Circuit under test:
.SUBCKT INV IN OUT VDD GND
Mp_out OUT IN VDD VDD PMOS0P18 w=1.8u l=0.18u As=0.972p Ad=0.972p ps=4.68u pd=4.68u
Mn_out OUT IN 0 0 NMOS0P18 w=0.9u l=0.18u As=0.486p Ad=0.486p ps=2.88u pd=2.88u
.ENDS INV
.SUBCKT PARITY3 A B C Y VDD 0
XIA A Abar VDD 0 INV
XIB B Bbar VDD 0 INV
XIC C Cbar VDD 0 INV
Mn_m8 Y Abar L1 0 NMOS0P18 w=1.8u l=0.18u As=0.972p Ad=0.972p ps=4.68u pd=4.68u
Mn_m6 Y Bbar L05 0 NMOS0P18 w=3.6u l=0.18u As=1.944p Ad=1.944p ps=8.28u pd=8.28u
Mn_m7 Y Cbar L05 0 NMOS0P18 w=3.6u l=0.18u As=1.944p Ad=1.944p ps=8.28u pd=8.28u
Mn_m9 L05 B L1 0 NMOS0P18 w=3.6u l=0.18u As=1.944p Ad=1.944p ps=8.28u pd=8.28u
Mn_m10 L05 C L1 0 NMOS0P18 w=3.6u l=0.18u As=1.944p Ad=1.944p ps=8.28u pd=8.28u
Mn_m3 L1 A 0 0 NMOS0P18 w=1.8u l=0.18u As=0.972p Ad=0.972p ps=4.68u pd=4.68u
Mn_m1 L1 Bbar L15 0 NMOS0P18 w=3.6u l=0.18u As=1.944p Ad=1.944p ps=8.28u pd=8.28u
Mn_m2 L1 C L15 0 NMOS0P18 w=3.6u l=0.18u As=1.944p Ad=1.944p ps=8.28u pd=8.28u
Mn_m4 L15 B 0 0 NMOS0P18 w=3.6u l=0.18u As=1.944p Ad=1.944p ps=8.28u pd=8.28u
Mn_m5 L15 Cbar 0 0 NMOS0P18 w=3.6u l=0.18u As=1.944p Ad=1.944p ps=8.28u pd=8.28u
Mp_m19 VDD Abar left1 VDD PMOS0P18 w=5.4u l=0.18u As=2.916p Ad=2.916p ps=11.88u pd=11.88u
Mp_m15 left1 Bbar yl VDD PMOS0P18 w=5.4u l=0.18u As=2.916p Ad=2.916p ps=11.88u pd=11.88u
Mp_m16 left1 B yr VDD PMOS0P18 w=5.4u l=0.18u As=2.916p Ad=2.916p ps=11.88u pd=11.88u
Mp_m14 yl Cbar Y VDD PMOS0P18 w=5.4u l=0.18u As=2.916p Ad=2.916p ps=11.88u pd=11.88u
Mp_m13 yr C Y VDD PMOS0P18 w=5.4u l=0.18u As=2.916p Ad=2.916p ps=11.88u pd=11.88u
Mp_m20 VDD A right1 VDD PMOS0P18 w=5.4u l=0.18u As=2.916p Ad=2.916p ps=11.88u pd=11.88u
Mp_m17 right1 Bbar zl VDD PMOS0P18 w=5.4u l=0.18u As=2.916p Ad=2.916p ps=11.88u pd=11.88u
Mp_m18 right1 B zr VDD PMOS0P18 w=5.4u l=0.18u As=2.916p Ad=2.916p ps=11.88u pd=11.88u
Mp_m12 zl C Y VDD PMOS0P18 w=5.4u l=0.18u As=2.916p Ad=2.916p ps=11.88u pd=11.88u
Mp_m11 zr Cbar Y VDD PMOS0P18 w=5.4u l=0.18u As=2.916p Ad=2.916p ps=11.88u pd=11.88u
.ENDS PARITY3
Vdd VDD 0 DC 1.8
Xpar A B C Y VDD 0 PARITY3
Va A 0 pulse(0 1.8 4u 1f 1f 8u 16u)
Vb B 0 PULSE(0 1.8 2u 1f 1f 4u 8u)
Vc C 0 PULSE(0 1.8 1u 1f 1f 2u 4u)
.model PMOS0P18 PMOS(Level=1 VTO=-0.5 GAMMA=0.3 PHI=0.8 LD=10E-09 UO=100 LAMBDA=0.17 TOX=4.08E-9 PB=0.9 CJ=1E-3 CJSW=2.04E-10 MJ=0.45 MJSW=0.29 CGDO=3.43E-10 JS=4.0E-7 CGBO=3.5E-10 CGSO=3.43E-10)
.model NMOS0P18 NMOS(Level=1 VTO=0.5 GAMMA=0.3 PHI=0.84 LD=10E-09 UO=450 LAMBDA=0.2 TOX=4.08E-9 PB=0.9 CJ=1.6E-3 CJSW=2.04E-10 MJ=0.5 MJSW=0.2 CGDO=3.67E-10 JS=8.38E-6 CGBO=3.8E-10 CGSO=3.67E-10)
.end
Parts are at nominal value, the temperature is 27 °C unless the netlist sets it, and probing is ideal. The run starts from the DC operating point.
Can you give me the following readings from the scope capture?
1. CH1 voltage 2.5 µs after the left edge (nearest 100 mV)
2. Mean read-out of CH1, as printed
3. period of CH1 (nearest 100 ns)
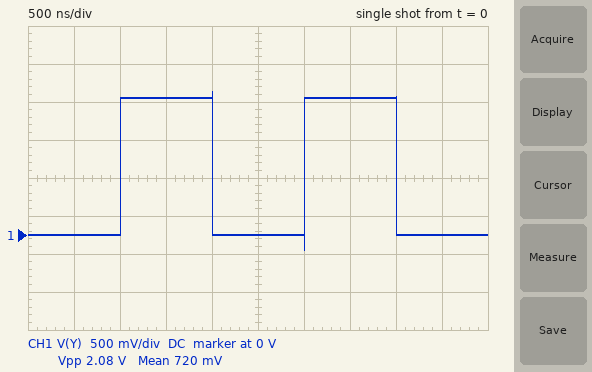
0 V
720 mV
2.0 µs
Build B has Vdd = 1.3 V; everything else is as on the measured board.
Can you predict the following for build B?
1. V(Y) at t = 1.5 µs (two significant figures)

1.3 V
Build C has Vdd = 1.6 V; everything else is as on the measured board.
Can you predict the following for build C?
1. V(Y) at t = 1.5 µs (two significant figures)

1.6 V
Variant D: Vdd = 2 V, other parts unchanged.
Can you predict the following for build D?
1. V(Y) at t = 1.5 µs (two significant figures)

2.0 V
